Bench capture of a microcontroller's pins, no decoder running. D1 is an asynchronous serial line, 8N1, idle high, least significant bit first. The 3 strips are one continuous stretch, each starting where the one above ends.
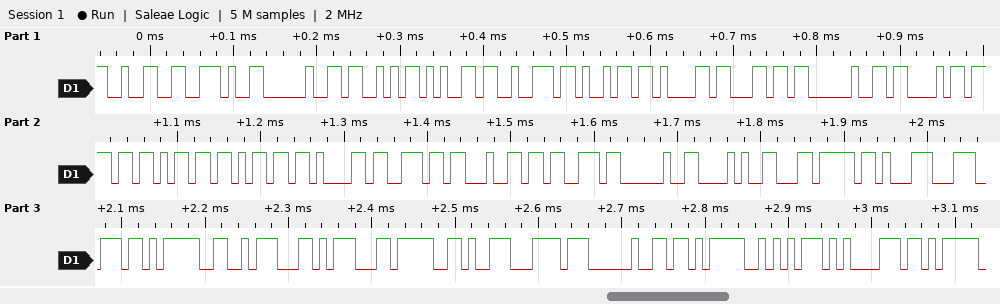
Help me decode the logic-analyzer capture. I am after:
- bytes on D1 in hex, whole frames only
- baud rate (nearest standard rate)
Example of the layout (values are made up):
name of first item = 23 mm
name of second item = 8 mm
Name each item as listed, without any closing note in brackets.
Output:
bytes on D1 in hex, whole frames only = 32 2E 20 53 65 72 69 61 6C 20 43 6F 6D 6D 61 6E 64 73 20 28 EC 8B 9C EB A6 AC EC 96 BC 20 EB AA 85 EB
baud rate = 115200 baud
